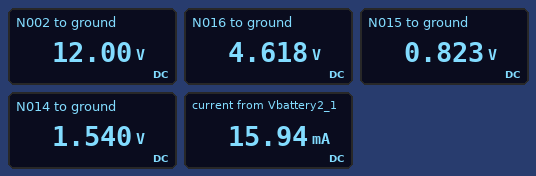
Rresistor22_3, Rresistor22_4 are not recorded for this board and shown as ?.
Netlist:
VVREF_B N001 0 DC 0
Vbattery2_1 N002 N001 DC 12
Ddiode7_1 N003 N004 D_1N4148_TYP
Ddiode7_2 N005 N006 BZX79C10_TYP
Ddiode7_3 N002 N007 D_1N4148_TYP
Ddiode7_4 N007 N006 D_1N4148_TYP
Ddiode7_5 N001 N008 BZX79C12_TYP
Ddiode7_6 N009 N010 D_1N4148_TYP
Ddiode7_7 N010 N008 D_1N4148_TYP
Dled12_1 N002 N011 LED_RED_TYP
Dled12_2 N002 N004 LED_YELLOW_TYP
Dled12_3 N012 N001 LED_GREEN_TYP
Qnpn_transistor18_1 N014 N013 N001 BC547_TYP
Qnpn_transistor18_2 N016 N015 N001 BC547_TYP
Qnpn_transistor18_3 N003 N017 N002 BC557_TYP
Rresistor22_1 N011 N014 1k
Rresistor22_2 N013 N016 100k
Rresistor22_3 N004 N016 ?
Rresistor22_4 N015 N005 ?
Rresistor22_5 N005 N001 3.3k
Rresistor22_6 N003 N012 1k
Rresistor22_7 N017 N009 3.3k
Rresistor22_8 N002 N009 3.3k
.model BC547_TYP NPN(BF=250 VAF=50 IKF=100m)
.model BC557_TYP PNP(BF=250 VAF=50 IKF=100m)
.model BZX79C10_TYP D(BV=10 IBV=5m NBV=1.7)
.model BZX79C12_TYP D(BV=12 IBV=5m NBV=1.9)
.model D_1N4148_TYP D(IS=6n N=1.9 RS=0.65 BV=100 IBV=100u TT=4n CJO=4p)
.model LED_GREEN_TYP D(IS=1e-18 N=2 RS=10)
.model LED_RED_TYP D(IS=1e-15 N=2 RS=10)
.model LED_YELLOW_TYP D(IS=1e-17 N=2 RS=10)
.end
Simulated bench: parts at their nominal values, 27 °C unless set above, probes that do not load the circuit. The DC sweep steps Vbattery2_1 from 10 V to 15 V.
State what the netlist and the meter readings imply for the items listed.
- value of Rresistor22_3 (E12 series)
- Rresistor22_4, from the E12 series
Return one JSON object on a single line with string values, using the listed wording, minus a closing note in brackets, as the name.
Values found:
{"value of Rresistor22_3": "820 Ω", "Rresistor22_4, from the E12 series": "8.2 kΩ"}
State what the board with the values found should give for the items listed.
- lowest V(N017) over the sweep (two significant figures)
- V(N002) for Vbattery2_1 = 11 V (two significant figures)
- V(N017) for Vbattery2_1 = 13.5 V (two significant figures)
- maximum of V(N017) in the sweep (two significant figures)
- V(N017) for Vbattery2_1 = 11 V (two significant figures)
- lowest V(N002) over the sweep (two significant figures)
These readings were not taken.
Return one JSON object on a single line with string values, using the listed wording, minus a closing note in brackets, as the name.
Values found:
{"lowest V(N017) over the sweep": "10 V", "V(N002) for Vbattery2_1 = 11 V": "11 V", "V(N017) for Vbattery2_1 = 13.5 V": "13 V", "maximum of V(N017) in the sweep": "14 V", "V(N017) for Vbattery2_1 = 11 V": "11 V", "lowest V(N002) over the sweep": "10 V"}
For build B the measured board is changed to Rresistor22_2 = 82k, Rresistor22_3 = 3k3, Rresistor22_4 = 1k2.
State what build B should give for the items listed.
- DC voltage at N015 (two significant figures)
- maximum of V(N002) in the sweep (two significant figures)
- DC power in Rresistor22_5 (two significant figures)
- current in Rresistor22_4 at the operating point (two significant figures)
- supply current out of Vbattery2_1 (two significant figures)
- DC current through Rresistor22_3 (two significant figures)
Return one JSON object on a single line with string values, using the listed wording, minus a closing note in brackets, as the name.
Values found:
{"DC voltage at N015": "810 mV", "maximum of V(N002) in the sweep": "15 V", "DC power in Rresistor22_5": "300 µW", "current in Rresistor22_4 at the operating point": "160 µA", "supply current out of Vbattery2_1": "3.5 mA", "DC current through Rresistor22_3": "3.1 mA"}
